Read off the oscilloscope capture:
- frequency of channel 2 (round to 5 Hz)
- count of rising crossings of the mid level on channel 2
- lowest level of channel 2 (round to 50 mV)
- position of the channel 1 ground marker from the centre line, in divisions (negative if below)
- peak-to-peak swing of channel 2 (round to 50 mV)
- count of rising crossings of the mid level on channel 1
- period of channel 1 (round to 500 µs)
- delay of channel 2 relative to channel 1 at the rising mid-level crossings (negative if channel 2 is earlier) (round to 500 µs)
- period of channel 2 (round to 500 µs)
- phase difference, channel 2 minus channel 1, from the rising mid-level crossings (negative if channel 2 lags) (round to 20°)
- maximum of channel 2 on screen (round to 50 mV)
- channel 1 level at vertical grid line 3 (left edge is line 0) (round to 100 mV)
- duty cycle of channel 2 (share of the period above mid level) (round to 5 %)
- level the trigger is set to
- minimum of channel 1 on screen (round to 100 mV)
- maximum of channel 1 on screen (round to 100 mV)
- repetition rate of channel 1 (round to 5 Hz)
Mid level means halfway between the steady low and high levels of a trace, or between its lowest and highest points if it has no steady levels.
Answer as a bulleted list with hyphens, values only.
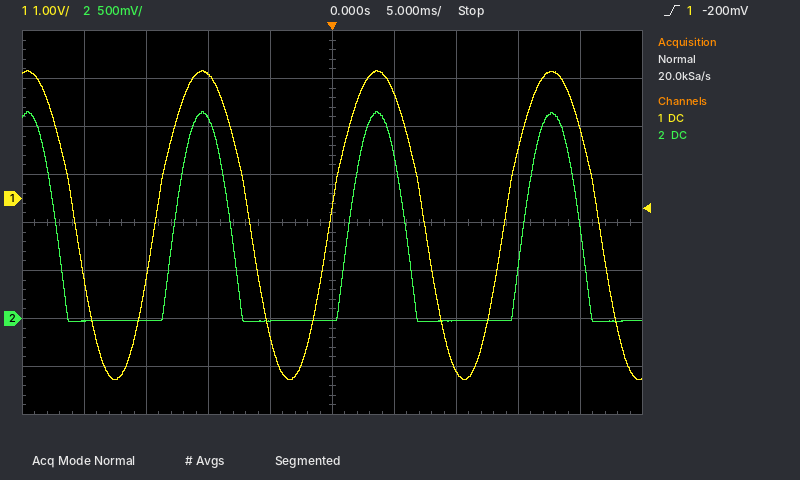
- 70 Hz
- 3
- -50 mV
- +0.5 div
- 2.20 V
- 3
- 14.0 ms
- +1.5 ms
- 14.0 ms
- -40°
- 2.15 V
- 2.6 V
- 30 %
- -200 mV
- -3.8 V
- 2.7 V
- 70 Hz
